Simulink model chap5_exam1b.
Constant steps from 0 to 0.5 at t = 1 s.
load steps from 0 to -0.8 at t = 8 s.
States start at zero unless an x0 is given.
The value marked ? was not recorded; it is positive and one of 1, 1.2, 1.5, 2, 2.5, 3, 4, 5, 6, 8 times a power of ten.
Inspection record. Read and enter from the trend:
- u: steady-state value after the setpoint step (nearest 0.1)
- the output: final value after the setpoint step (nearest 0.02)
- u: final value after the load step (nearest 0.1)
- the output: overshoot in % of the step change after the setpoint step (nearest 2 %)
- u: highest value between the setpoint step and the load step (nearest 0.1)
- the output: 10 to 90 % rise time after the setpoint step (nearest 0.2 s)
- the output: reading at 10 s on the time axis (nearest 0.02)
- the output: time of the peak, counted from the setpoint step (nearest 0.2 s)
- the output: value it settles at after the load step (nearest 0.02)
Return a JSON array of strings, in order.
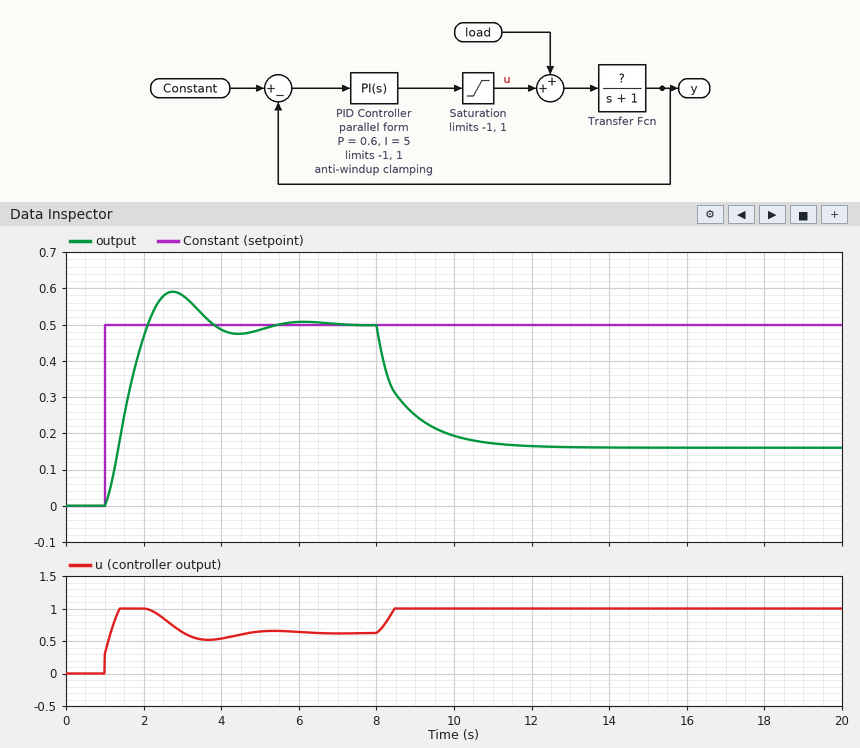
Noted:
["0.6", "0.50", "1.0", "18 %", "1.0", "0.8 s", "0.20", "1.8 s", "0.16"]
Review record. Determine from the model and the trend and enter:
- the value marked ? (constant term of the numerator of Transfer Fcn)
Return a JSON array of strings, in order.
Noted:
["0.8"]
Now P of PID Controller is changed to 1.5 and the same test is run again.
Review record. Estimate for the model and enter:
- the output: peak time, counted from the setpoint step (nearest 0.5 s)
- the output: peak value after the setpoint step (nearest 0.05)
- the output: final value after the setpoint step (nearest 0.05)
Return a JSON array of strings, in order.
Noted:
["1.5 s", "0.55", "0.50"]
